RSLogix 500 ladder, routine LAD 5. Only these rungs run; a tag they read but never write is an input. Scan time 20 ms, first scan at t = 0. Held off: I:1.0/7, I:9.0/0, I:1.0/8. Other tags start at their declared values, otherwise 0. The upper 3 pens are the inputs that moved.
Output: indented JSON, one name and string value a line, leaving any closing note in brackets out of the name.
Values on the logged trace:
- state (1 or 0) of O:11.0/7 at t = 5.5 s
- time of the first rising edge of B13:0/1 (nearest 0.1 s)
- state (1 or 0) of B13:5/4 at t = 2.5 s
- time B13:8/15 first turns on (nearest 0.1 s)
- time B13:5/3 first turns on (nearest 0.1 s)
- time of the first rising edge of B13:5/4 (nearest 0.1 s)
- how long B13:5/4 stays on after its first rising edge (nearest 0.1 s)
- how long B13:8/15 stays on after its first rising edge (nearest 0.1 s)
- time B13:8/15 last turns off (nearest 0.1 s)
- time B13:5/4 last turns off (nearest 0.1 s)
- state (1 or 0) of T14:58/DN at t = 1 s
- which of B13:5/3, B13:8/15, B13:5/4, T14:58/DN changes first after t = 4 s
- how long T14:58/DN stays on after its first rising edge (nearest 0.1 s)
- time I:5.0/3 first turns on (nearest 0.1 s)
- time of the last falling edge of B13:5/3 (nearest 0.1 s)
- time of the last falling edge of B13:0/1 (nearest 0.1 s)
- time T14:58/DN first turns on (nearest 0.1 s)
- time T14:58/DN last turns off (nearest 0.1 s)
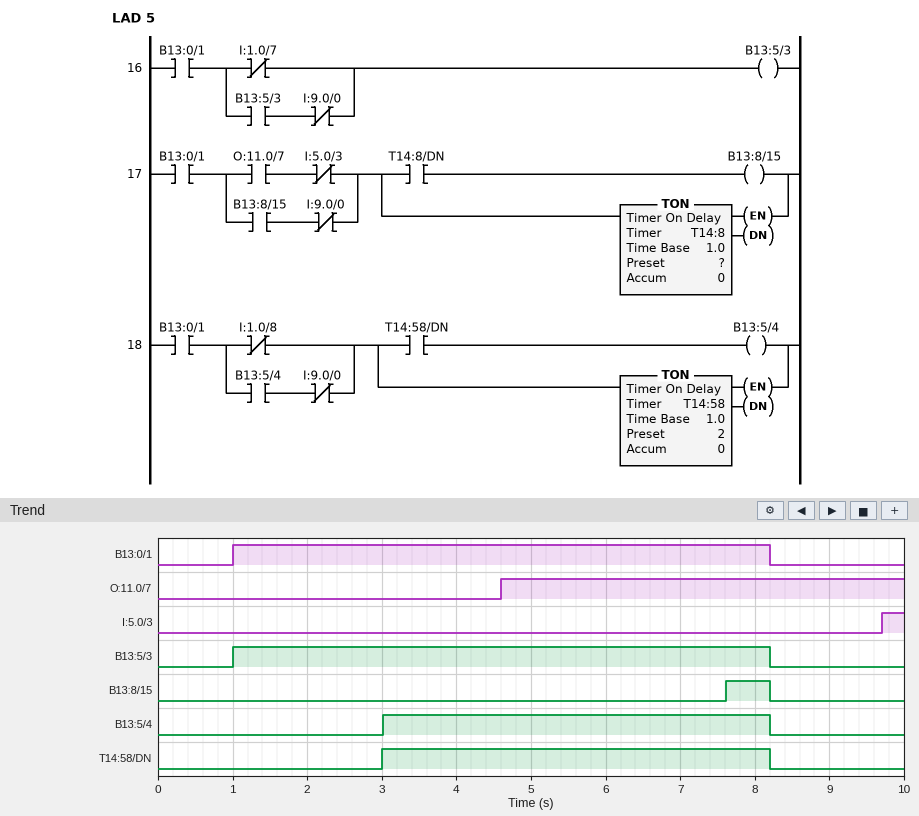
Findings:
{
  "state (1 or 0) of O:11.0/7 at t = 5.5 s": "1",
  "time of the first rising edge of B13:0/1": "1.0 s",
  "state (1 or 0) of B13:5/4 at t = 2.5 s": "0",
  "time B13:8/15 first turns on": "7.6 s",
  "time B13:5/3 first turns on": "1.0 s",
  "time of the first rising edge of B13:5/4": "3.0 s",
  "how long B13:5/4 stays on after its first rising edge": "5.2 s",
  "how long B13:8/15 stays on after its first rising edge": "0.6 s",
  "time B13:8/15 last turns off": "8.2 s",
  "time B13:5/4 last turns off": "8.2 s",
  "state (1 or 0) of T14:58/DN at t = 1 s": "0",
  "which of B13:5/3, B13:8/15, B13:5/4, T14:58/DN changes first after t = 4 s": "B13:8/15",
  "how long T14:58/DN stays on after its first rising edge": "5.2 s",
  "time I:5.0/3 first turns on": "9.7 s",
  "time of the last falling edge of B13:5/3": "8.2 s",
  "time of the last falling edge of B13:0/1": "8.2 s",
  "time T14:58/DN first turns on": "3.0 s",
  "time T14:58/DN last turns off": "8.2 s"
}
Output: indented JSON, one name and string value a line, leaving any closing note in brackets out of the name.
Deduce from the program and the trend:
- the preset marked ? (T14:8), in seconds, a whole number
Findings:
{
  "the preset marked ? (T14:8), in seconds, a whole number": "3 s"
}
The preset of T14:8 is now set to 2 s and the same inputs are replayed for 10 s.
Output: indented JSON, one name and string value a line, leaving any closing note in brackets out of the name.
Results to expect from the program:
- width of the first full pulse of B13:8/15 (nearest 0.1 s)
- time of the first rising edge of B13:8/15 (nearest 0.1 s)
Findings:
{
  "width of the first full pulse of B13:8/15": "1.6 s",
  "time of the first rising edge of B13:8/15": "6.6 s"
}
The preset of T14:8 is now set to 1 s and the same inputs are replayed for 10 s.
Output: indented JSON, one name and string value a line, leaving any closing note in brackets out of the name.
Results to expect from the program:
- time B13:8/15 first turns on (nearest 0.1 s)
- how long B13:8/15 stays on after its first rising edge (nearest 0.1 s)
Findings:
{
  "time B13:8/15 first turns on": "5.6 s",
  "how long B13:8/15 stays on after its first rising edge": "2.6 s"
}
